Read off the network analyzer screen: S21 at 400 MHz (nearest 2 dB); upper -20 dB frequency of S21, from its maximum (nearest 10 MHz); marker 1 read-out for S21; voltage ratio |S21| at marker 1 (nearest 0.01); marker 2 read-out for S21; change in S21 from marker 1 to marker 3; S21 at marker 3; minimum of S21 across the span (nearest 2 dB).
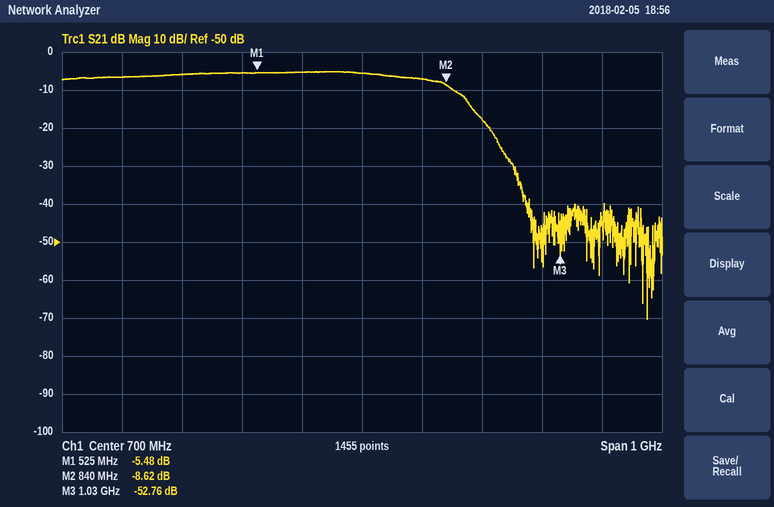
-6 dB
930 MHz
-5.48 dB
0.53
-8.62 dB
-47.28 dB
-52.76 dB
-70 dB
